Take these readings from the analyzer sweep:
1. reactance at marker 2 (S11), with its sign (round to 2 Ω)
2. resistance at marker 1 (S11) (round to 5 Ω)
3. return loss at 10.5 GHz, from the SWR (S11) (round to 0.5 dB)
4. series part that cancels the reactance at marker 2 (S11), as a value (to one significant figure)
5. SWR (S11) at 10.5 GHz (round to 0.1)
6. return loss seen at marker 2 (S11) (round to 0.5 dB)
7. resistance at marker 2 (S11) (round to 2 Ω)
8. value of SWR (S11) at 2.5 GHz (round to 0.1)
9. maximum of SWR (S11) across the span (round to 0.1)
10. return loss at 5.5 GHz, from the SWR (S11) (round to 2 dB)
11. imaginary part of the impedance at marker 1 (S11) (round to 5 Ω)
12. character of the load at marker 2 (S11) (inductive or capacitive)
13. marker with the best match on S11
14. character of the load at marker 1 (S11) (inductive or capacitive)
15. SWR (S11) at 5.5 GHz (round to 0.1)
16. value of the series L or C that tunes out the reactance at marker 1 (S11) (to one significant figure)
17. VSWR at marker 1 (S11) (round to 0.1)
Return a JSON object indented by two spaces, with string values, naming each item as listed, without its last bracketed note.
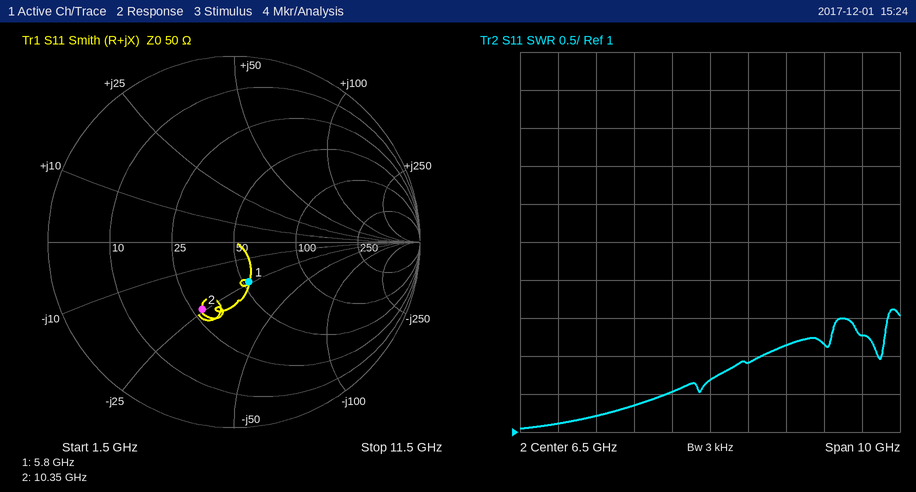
{
  "reactance at marker 2 (S11), with its sign": "-24 Ω",
  "resistance at marker 1 (S11)": "55 Ω",
  "return loss at 10.5 GHz, from the SWR (S11)": "8.0 dB",
  "series part that cancels the reactance at marker 2 (S11), as a value": "400 pH",
  "SWR (S11) at 10.5 GHz": "2.3",
  "return loss seen at marker 2 (S11)": "8.0 dB",
  "resistance at marker 2 (S11)": "28 Ω",
  "value of SWR (S11) at 2.5 GHz": "1.1",
  "maximum of SWR (S11) across the span": "2.6",
  "return loss at 5.5 GHz, from the SWR (S11)": "14 dB",
  "imaginary part of the impedance at marker 1 (S11)": "-25 Ω",
  "character of the load at marker 2 (S11)": "capacitive",
  "marker with the best match on S11": "marker 1",
  "character of the load at marker 1 (S11)": "capacitive",
  "SWR (S11) at 5.5 GHz": "1.5",
  "value of the series L or C that tunes out the reactance at marker 1 (S11)": "700 pH",
  "VSWR at marker 1 (S11)": "1.6"
}
